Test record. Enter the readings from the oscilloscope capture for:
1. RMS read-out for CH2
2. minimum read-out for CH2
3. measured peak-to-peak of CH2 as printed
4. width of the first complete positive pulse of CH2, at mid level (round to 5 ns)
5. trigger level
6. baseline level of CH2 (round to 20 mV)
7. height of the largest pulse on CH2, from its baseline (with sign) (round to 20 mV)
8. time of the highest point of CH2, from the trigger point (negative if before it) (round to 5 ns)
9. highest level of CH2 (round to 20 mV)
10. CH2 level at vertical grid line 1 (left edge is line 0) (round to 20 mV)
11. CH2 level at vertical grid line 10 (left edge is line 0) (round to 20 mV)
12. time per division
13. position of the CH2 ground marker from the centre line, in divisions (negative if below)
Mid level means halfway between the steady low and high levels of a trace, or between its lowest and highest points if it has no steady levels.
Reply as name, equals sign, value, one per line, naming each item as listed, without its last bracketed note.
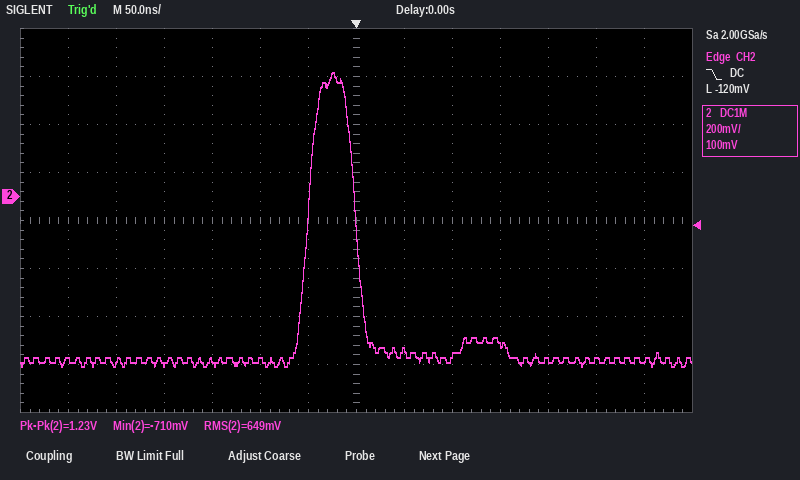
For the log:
RMS read-out for CH2 = 649 mV
minimum read-out for CH2 = -710 mV
measured peak-to-peak of CH2 as printed = 1.23 V
width of the first complete positive pulse of CH2, at mid level = 50 ns
trigger level = -120 mV
baseline level of CH2 = -680 mV
height of the largest pulse on CH2, from its baseline (with sign) = +1.20 V
time of the highest point of CH2, from the trigger point (negative if before it) = -25 ns
highest level of CH2 = 520 mV
CH2 level at vertical grid line 1 (left edge is line 0) = -680 mV
CH2 level at vertical grid line 10 (left edge is line 0) = -620 mV
time per division = 50 ns
position of the CH2 ground marker from the centre line, in divisions = +0.5 div
